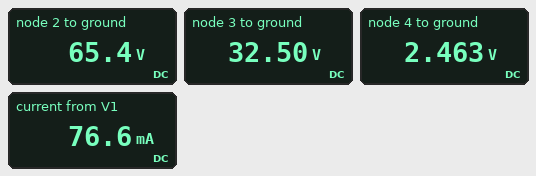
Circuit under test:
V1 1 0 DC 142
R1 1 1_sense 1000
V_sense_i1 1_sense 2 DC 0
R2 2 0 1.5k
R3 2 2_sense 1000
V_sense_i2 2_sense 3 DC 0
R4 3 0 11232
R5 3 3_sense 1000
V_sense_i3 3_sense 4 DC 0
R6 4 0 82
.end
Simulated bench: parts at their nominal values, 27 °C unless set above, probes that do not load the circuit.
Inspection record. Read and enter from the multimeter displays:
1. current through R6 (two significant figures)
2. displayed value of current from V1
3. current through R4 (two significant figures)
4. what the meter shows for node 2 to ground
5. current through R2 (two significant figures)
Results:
30 mA
76.6 mA
2.9 mA
65.4 V
44 mA
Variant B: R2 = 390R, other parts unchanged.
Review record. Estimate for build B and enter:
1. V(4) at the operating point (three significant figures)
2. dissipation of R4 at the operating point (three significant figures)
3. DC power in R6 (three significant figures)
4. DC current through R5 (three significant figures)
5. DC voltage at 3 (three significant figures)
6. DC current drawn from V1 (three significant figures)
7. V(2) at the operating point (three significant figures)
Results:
1.31 V
26.8 mW
21.1 mW
16.0 mA
17.3 V
107 mA
34.9 V
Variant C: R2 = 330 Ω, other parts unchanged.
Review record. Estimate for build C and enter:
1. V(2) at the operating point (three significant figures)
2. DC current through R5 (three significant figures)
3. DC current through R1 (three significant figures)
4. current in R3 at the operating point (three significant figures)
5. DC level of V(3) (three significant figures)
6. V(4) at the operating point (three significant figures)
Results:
31.3 V
14.4 mA
111 mA
15.8 mA
15.6 V
1.18 V
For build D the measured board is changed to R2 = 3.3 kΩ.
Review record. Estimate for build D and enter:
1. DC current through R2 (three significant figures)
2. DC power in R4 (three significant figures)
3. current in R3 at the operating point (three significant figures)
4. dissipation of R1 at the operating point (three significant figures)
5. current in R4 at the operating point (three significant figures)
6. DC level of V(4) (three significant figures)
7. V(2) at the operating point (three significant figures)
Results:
23.8 mA
136 mW
39.6 mA
4.02 W
3.48 mA
2.96 V
78.6 V
